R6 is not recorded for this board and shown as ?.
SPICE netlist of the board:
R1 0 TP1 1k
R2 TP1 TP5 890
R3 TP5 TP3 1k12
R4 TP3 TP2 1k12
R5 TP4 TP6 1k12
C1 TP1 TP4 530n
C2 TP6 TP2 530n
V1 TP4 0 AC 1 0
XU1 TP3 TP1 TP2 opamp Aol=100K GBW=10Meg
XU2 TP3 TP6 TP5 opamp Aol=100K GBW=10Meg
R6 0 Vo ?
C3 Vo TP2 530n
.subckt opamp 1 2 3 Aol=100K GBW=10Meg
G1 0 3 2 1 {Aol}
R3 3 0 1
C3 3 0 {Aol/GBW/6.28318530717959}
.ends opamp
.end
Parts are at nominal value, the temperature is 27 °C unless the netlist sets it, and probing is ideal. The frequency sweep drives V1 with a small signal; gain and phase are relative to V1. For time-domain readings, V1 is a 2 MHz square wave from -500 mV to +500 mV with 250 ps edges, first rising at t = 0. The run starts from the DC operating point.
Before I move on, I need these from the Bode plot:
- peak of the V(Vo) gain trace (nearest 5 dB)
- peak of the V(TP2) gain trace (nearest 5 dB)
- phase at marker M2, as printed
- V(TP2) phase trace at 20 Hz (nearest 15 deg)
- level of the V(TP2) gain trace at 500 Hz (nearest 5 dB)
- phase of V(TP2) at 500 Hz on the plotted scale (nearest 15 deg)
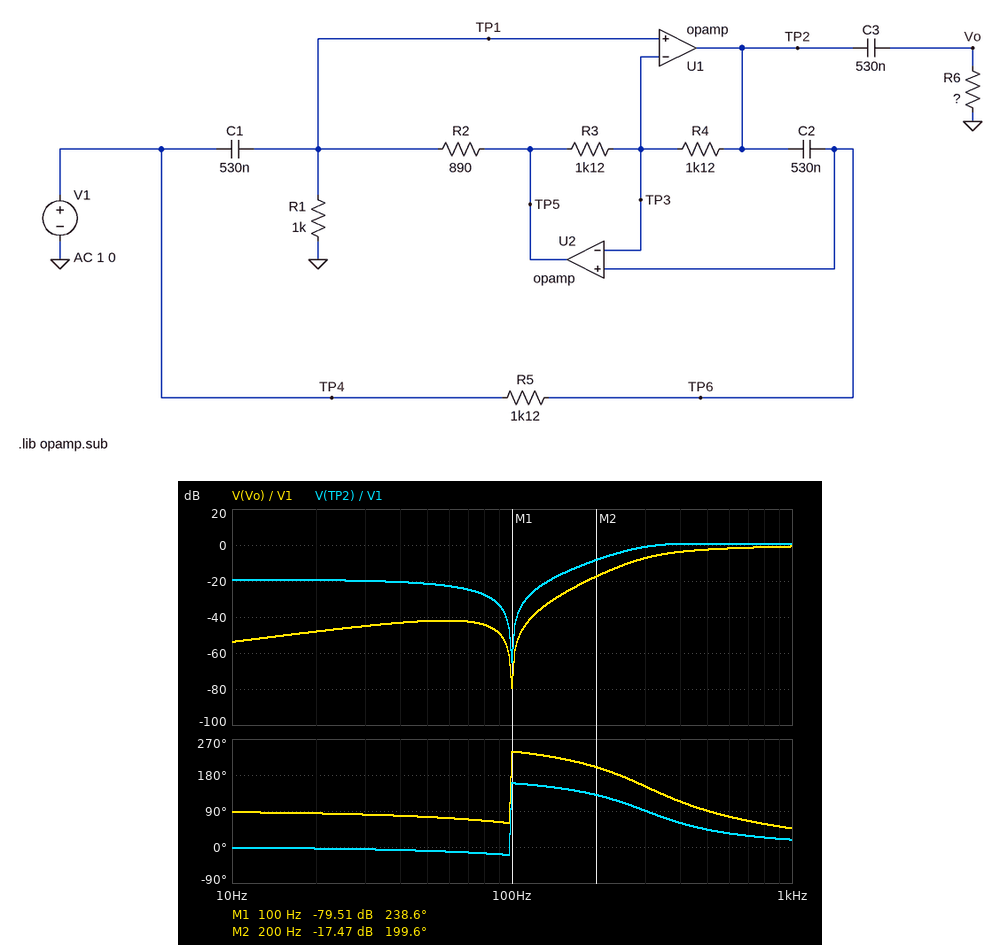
0 dB
0 dB
199.6 deg
0 deg
0 dB
45 deg
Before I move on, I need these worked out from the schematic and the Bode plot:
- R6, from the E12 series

560 Ω
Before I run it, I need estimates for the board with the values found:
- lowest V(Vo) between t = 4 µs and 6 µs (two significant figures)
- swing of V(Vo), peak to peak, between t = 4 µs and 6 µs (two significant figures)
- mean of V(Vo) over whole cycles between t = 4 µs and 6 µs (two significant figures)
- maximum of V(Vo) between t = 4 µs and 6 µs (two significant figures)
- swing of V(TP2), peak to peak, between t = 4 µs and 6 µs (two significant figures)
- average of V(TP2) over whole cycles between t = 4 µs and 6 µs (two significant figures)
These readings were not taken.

-220 mV
1.4 V
490 mV
1.2 V
1.4 V
440 mV
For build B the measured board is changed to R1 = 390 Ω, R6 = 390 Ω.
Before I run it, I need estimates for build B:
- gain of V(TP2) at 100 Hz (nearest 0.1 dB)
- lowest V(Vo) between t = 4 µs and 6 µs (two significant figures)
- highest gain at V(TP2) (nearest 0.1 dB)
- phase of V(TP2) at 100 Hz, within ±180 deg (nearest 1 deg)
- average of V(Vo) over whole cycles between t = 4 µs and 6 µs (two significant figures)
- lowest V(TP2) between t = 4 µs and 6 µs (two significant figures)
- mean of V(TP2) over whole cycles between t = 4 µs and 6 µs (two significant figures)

1.1 dB
-240 mV
2.2 dB
136 deg
480 mV
420 mV
1.1 V
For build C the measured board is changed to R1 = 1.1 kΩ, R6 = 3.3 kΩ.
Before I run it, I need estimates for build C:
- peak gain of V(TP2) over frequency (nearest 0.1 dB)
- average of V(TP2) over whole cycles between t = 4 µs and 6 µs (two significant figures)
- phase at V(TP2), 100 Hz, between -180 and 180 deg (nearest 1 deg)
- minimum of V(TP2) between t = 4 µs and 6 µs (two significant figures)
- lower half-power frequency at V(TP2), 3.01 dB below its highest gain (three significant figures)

0.9 dB
400 mV
-19 deg
-310 mV
280 Hz
